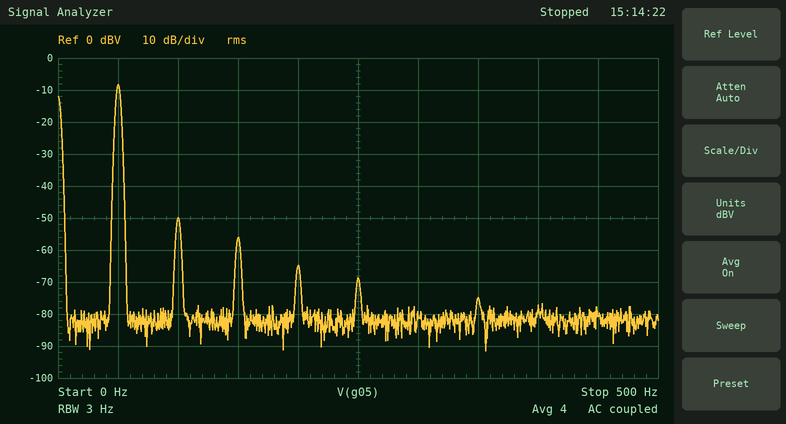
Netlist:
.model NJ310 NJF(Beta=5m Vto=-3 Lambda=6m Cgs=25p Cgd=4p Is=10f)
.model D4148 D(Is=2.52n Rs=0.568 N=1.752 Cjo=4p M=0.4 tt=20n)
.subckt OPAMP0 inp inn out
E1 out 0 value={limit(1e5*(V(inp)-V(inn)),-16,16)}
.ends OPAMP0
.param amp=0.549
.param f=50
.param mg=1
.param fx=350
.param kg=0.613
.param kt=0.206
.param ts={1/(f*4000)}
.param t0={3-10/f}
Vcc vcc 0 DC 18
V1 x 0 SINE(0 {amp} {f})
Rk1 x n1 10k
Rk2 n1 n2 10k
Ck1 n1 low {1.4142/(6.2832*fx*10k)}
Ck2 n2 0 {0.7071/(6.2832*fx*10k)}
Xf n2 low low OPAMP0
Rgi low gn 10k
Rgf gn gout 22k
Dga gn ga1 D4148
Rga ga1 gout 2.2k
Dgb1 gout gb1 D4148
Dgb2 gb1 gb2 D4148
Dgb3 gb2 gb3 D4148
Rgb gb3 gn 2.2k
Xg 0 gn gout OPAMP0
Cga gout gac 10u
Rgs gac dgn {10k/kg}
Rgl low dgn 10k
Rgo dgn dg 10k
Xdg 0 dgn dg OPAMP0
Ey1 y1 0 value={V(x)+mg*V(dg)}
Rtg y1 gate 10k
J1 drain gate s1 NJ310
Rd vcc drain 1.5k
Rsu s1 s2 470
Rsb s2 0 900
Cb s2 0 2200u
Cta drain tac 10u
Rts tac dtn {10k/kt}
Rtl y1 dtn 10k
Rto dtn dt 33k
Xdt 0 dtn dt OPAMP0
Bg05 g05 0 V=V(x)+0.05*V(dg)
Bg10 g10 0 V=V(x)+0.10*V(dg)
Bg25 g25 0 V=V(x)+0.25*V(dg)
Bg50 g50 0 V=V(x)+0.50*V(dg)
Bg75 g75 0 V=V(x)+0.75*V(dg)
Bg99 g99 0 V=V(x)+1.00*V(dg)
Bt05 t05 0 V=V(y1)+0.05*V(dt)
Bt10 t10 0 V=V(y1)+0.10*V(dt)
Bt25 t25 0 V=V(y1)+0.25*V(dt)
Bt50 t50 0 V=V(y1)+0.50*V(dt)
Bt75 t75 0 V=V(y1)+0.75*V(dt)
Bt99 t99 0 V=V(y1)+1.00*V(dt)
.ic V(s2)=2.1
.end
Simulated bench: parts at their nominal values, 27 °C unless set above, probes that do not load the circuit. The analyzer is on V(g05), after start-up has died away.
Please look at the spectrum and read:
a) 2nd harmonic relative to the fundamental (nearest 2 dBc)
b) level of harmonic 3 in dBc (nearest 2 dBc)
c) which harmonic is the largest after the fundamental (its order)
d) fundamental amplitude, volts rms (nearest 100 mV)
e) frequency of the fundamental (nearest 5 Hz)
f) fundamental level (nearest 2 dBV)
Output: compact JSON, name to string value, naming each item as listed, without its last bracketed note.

{"2nd harmonic relative to the fundamental": "-42 dBc", "level of harmonic 3 in dBc": "-48 dBc", "which harmonic is the largest after the fundamental": "2", "fundamental amplitude, volts rms": "400 mV", "frequency of the fundamental": "50 Hz", "fundamental level": "-8 dBV"}
